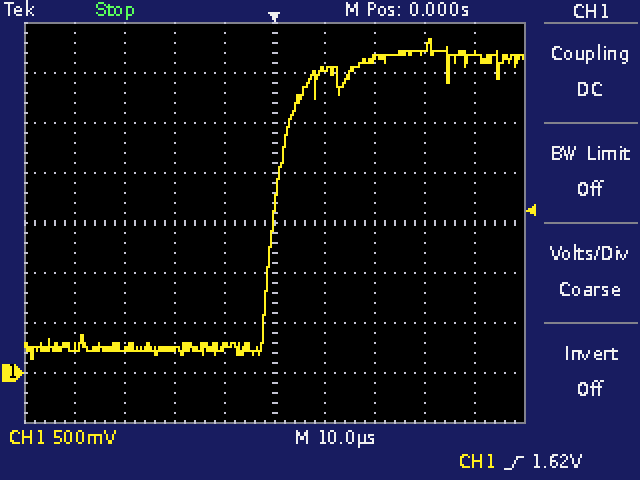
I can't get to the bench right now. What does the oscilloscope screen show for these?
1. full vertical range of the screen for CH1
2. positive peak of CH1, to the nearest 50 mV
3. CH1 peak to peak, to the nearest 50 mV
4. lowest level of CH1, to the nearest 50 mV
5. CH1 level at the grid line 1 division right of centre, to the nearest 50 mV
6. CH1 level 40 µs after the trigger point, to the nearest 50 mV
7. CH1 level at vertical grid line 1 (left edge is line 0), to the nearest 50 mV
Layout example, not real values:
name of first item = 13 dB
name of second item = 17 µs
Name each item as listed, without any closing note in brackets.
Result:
full vertical range of the screen for CH1 = 4 V
positive peak of CH1, to the nearest 50 mV = 3.35 V
CH1 peak to peak, to the nearest 50 mV = 3.20 V
lowest level of CH1, to the nearest 50 mV = 150 mV
CH1 level at the grid line 1 division right of centre, to the nearest 50 mV = 3.05 V
CH1 level 40 µs after the trigger point, to the nearest 50 mV = 3.20 V
CH1 level at vertical grid line 1 (left edge is line 0), to the nearest 50 mV = 250 mV
